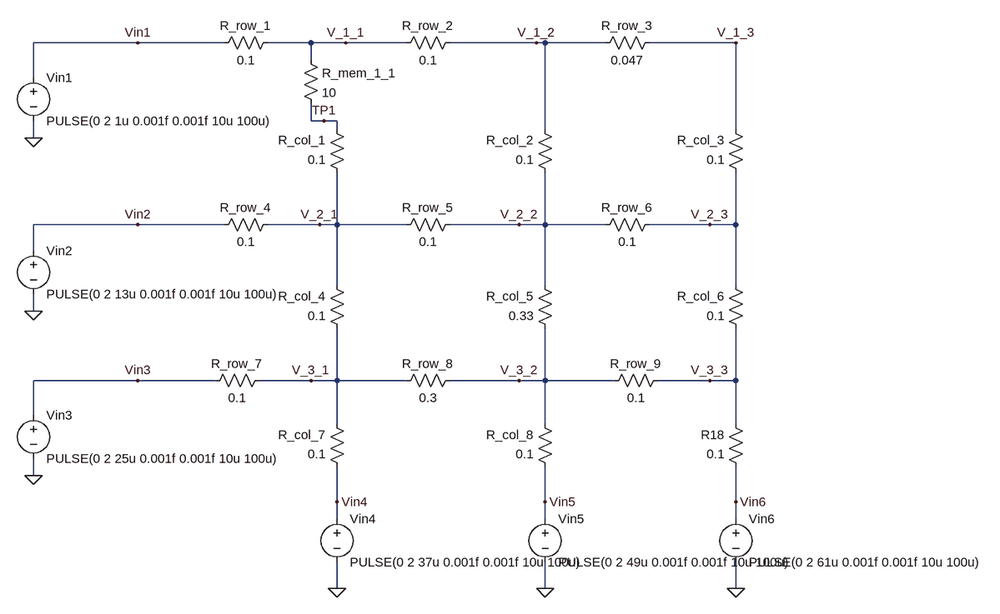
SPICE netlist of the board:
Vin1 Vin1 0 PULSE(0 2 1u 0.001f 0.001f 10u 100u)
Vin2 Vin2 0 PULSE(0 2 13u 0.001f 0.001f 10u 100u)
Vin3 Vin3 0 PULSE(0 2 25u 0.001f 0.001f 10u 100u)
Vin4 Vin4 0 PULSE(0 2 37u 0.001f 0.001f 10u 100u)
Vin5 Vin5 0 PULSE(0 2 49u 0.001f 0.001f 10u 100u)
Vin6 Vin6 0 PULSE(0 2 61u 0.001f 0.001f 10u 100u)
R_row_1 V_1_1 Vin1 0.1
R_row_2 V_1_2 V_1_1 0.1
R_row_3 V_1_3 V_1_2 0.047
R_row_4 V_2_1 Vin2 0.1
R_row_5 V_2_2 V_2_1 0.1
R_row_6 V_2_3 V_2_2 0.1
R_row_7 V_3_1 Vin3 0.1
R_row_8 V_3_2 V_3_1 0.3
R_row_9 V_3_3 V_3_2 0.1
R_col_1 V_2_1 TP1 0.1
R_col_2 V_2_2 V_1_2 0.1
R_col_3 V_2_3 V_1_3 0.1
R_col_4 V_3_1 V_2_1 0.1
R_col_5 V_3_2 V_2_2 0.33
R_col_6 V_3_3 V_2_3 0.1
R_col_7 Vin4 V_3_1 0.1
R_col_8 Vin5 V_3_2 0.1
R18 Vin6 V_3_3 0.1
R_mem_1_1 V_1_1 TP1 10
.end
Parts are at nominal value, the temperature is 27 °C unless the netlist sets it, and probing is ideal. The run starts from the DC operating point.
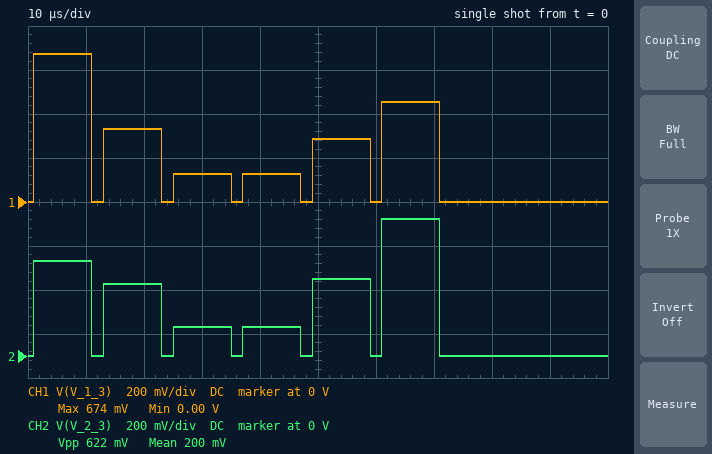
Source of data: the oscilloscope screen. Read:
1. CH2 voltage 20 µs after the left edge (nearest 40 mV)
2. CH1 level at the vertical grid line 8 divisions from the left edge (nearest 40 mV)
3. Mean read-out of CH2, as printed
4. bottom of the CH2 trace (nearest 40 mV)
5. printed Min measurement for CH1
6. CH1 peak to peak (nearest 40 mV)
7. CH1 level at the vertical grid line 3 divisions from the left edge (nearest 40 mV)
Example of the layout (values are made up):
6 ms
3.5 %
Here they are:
320 mV
0 V
200 mV
0 V
0.00 V
680 mV
120 mV
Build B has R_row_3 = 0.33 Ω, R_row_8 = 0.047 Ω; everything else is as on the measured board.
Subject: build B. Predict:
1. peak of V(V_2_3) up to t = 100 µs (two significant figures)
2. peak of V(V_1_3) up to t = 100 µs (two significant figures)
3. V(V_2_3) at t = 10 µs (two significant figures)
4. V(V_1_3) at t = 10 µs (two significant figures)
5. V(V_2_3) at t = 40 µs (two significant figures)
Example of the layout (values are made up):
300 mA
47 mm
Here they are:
640 mV
560 mV
350 mV
470 mV
190 mV
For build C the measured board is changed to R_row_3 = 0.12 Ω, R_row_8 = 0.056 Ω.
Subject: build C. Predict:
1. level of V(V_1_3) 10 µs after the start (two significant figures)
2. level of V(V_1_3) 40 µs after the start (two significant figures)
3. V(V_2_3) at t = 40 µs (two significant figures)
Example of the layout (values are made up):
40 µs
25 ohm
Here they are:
590 mV
170 mV
180 mV
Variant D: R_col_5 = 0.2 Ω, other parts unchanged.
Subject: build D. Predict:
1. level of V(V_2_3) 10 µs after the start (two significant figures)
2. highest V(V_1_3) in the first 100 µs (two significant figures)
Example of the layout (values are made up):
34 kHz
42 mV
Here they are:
420 mV
660 mV
